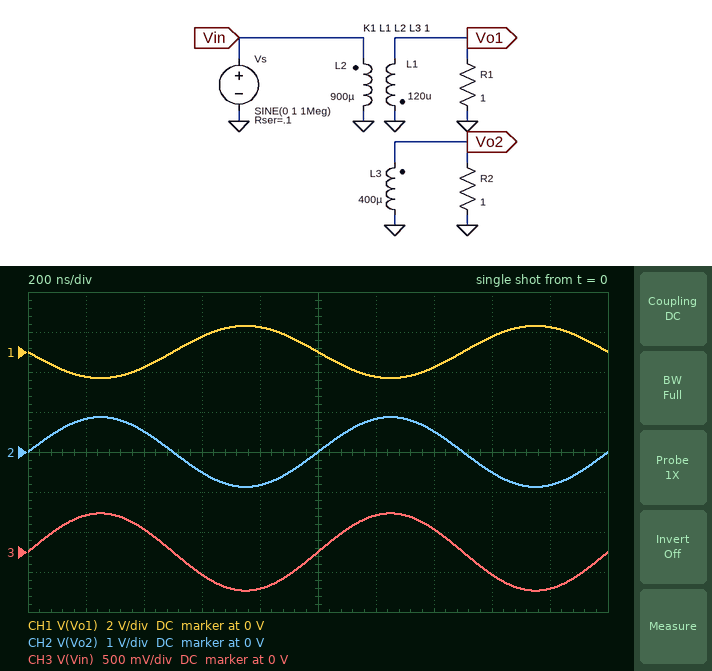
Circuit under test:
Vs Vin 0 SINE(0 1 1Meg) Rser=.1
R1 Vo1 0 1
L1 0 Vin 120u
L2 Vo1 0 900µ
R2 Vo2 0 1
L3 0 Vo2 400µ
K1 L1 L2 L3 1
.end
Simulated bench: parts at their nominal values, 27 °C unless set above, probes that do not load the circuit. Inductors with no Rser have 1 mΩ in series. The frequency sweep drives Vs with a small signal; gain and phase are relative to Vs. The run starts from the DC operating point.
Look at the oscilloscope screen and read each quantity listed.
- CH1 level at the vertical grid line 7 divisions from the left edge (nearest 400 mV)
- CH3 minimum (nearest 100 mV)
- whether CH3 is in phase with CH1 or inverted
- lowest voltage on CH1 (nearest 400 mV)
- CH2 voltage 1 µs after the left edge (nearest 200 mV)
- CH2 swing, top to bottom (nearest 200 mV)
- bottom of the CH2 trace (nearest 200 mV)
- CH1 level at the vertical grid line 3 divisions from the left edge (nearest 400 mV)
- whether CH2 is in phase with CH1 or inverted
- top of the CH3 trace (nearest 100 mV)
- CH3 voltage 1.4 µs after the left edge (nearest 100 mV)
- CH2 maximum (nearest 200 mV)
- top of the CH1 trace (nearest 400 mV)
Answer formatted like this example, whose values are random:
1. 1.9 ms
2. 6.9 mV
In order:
1. -800 mV
2. -500 mV
3. inverted
4. -1.2 V
5. 0 V
6. 1.8 V
7. -800 mV
8. 800 mV
9. inverted
10. 500 mV
11. 300 mV
12. 800 mV
13. 1.2 V
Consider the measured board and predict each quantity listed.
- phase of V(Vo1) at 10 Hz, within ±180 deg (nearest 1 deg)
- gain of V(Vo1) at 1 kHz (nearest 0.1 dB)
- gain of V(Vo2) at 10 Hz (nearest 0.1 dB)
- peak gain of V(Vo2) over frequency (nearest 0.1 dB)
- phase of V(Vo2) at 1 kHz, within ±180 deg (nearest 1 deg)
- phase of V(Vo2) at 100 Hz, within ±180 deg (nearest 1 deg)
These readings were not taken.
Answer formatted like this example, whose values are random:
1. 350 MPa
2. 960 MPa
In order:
1. -99 deg
2. 2.3 dB
3. -17.4 dB
4. -1.2 dB
5. 4 deg
6. 33 deg
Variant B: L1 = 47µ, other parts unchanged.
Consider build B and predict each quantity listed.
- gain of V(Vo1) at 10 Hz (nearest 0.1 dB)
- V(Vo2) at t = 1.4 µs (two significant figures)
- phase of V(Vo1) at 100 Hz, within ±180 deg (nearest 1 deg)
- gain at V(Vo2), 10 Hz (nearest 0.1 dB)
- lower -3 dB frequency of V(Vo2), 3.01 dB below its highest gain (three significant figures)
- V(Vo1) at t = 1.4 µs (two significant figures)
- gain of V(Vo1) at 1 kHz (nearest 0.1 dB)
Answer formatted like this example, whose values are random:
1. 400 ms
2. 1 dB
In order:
1. -17.9 dB
2. 450 mV
3. -138 deg
4. -21.4 dB
5. 90.2 Hz
6. -680 mV
7. 1.2 dB
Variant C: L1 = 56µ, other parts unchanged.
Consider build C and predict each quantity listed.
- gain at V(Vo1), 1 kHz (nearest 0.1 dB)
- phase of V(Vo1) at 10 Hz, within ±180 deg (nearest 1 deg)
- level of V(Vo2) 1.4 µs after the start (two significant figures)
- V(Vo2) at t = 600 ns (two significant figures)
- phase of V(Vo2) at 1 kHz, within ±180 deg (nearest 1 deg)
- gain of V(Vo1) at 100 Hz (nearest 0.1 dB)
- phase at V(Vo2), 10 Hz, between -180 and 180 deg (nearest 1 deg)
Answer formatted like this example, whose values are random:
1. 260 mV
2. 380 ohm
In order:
1. 1.5 dB
2. -97 deg
3. 470 mV
4. -470 mV
5. 5 deg
6. -0.8 dB
7. 83 deg
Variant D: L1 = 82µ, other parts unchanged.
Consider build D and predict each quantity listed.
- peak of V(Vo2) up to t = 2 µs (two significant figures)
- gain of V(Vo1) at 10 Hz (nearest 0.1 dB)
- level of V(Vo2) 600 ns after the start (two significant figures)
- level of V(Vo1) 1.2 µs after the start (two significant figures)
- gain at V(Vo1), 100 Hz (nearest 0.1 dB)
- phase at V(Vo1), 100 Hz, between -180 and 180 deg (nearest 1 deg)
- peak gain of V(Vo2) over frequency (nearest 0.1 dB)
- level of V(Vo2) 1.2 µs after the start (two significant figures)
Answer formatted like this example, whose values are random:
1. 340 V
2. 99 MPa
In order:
1. 850 mV
2. -15.5 dB
3. -500 mV
4. -1.2 V
5. 0.1 dB
6. -143 deg
7. -1.4 dB
8. 810 mV
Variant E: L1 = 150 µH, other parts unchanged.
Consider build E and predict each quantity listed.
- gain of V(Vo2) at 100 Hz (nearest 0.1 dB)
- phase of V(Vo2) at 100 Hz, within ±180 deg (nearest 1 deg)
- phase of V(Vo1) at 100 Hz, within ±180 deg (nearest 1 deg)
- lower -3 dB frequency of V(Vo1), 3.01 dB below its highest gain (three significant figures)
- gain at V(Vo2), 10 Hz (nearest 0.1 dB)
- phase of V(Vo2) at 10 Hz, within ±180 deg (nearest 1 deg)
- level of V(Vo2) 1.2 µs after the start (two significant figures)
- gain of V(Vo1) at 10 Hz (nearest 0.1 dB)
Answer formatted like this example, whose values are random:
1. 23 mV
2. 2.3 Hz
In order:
1. -2.4 dB
2. 30 deg
3. -150 deg
4. 57.2 Hz
5. -16.5 dB
6. 80 deg
7. 830 mV
8. -13.0 dB
